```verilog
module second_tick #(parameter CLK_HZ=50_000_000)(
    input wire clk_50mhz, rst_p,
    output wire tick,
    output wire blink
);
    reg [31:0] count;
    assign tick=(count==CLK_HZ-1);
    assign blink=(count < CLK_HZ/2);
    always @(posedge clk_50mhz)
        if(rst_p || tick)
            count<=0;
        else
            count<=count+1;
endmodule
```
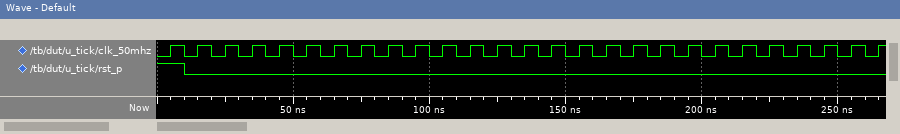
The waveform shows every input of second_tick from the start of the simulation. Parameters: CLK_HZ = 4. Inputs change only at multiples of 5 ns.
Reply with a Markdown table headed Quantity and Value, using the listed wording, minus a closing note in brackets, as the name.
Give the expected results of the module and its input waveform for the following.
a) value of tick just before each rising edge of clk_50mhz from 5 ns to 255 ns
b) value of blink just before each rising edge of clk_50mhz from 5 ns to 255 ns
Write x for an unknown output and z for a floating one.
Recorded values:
| Quantity | Value |
|---|---|
| value of tick just before each rising edge of clk_50mhz from 5 ns to 255 ns | x 0 0 0 1 0 0 0 1 0 0 0 1 0 0 0 1 0 0 0 1 0 0 0 1 0 |
| value of blink just before each rising edge of clk_50mhz from 5 ns to 255 ns | x 1 1 0 0 1 1 0 0 1 1 0 0 1 1 0 0 1 1 0 0 1 1 0 0 1 |
